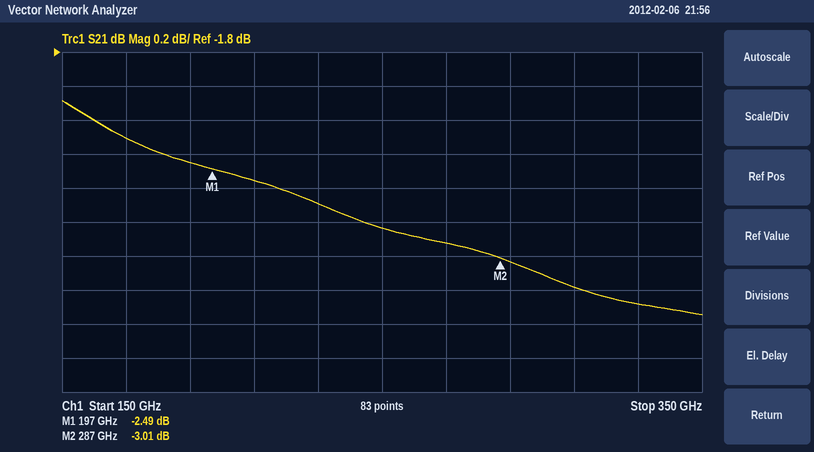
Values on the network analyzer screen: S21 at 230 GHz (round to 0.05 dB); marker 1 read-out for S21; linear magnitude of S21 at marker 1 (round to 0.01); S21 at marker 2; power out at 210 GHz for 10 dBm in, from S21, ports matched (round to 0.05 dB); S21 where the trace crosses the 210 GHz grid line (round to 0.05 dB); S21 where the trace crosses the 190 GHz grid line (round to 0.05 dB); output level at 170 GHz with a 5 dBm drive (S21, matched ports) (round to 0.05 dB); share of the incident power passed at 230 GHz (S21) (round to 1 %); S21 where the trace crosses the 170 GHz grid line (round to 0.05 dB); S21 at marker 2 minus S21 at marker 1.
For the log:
-2.70 dB
-2.49 dB
0.75
-3.01 dB
7.45 dBm
-2.55 dB
-2.45 dB
2.70 dBm
54 %
-2.30 dB
-0.52 dB
